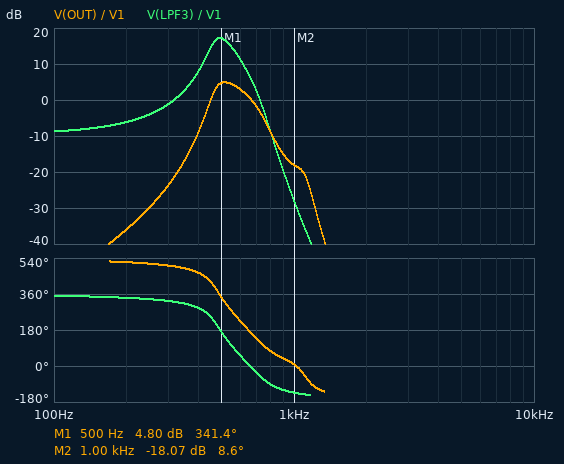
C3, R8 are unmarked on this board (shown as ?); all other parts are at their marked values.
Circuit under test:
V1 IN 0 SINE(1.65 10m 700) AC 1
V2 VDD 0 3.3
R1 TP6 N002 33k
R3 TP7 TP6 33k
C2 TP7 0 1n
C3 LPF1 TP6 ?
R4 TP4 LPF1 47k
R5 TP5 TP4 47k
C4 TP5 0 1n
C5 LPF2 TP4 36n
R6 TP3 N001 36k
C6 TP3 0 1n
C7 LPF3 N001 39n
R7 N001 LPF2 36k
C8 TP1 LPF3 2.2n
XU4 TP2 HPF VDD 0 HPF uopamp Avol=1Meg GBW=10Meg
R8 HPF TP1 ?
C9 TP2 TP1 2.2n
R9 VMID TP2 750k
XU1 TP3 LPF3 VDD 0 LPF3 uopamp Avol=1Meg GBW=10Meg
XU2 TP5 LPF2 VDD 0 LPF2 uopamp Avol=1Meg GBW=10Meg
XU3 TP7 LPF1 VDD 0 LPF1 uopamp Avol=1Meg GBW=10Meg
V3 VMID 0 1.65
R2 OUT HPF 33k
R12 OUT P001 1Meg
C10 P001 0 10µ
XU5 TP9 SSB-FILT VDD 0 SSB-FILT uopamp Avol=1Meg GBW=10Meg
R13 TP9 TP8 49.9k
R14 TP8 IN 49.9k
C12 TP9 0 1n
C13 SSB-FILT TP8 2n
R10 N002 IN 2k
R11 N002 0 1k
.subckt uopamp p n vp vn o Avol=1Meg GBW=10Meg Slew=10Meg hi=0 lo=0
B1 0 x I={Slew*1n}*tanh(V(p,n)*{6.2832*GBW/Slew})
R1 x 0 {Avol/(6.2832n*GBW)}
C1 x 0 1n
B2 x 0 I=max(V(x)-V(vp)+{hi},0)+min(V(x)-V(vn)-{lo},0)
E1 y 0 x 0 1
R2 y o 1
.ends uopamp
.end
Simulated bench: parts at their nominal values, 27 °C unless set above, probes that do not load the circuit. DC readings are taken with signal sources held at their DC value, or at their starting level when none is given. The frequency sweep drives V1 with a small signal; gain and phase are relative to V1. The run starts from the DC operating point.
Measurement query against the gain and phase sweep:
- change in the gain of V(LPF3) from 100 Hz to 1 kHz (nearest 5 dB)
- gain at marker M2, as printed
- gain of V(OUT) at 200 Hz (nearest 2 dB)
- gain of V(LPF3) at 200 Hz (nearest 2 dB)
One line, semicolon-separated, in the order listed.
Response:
-20 dB; -18.07 dB; -36 dB; -6 dB
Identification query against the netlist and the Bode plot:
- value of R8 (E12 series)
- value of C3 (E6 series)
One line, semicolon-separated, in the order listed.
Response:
5.6 kΩ; 100 nF
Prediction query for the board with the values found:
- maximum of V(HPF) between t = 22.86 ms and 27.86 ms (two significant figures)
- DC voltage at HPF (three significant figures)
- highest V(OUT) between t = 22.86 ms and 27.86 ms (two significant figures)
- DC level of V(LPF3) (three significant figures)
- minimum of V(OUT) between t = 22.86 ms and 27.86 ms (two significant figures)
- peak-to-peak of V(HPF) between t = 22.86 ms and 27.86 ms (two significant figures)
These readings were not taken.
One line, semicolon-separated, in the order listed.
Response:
1.7 V; 1.65 V; 1.7 V; 550 mV; 1.6 V; 17 mV
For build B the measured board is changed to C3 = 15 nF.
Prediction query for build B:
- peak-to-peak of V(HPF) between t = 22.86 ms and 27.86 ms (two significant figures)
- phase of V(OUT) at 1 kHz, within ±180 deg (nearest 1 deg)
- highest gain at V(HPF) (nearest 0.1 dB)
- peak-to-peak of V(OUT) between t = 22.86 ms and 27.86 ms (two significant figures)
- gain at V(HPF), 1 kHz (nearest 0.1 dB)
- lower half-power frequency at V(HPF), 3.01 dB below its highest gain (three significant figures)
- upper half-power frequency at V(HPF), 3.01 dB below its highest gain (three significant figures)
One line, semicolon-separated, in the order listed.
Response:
27 mV; 131 deg; 2.6 dB; 26 mV; -1.8 dB; 568 Hz; 816 Hz
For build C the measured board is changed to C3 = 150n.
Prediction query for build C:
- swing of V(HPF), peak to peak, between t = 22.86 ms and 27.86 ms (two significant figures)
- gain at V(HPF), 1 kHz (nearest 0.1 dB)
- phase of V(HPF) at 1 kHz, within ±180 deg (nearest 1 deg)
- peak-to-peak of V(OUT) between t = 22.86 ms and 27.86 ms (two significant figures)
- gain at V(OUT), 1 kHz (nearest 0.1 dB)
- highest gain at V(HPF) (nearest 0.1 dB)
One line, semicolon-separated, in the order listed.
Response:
8.8 mV; -22.1 dB; 6 deg; 8.5 mV; -22.4 dB; -2.9 dB
